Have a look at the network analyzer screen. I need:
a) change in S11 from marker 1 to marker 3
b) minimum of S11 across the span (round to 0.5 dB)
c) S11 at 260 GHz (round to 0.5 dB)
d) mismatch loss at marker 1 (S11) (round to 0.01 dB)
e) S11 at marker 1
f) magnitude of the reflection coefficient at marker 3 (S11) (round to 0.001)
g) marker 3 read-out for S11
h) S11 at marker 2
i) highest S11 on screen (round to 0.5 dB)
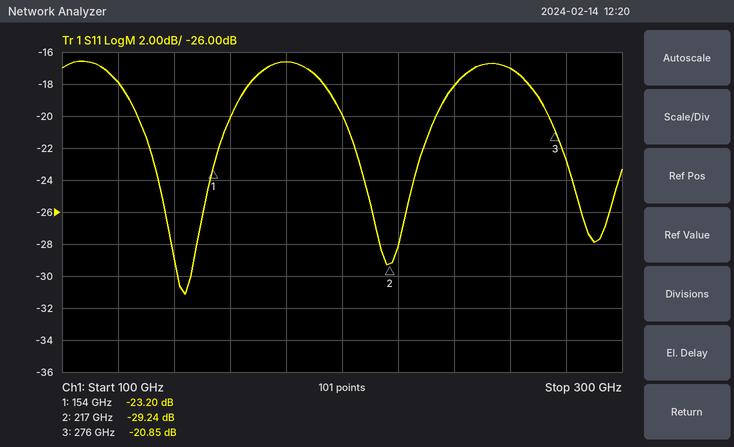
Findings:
2.35 dB
-31.0 dB
-17.0 dB
0.02 dB
-23.20 dB
0.091
-20.85 dB
-29.24 dB
-16.5 dB
